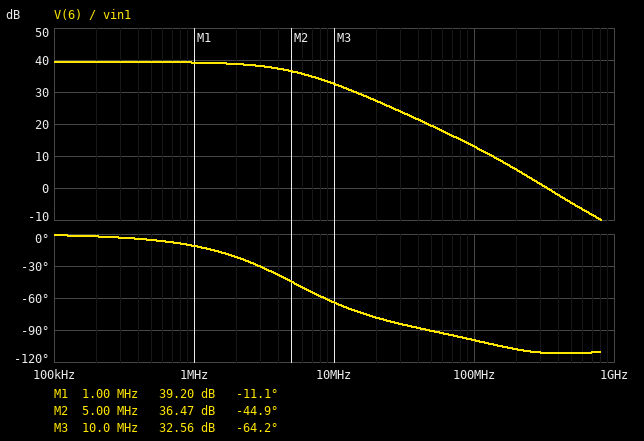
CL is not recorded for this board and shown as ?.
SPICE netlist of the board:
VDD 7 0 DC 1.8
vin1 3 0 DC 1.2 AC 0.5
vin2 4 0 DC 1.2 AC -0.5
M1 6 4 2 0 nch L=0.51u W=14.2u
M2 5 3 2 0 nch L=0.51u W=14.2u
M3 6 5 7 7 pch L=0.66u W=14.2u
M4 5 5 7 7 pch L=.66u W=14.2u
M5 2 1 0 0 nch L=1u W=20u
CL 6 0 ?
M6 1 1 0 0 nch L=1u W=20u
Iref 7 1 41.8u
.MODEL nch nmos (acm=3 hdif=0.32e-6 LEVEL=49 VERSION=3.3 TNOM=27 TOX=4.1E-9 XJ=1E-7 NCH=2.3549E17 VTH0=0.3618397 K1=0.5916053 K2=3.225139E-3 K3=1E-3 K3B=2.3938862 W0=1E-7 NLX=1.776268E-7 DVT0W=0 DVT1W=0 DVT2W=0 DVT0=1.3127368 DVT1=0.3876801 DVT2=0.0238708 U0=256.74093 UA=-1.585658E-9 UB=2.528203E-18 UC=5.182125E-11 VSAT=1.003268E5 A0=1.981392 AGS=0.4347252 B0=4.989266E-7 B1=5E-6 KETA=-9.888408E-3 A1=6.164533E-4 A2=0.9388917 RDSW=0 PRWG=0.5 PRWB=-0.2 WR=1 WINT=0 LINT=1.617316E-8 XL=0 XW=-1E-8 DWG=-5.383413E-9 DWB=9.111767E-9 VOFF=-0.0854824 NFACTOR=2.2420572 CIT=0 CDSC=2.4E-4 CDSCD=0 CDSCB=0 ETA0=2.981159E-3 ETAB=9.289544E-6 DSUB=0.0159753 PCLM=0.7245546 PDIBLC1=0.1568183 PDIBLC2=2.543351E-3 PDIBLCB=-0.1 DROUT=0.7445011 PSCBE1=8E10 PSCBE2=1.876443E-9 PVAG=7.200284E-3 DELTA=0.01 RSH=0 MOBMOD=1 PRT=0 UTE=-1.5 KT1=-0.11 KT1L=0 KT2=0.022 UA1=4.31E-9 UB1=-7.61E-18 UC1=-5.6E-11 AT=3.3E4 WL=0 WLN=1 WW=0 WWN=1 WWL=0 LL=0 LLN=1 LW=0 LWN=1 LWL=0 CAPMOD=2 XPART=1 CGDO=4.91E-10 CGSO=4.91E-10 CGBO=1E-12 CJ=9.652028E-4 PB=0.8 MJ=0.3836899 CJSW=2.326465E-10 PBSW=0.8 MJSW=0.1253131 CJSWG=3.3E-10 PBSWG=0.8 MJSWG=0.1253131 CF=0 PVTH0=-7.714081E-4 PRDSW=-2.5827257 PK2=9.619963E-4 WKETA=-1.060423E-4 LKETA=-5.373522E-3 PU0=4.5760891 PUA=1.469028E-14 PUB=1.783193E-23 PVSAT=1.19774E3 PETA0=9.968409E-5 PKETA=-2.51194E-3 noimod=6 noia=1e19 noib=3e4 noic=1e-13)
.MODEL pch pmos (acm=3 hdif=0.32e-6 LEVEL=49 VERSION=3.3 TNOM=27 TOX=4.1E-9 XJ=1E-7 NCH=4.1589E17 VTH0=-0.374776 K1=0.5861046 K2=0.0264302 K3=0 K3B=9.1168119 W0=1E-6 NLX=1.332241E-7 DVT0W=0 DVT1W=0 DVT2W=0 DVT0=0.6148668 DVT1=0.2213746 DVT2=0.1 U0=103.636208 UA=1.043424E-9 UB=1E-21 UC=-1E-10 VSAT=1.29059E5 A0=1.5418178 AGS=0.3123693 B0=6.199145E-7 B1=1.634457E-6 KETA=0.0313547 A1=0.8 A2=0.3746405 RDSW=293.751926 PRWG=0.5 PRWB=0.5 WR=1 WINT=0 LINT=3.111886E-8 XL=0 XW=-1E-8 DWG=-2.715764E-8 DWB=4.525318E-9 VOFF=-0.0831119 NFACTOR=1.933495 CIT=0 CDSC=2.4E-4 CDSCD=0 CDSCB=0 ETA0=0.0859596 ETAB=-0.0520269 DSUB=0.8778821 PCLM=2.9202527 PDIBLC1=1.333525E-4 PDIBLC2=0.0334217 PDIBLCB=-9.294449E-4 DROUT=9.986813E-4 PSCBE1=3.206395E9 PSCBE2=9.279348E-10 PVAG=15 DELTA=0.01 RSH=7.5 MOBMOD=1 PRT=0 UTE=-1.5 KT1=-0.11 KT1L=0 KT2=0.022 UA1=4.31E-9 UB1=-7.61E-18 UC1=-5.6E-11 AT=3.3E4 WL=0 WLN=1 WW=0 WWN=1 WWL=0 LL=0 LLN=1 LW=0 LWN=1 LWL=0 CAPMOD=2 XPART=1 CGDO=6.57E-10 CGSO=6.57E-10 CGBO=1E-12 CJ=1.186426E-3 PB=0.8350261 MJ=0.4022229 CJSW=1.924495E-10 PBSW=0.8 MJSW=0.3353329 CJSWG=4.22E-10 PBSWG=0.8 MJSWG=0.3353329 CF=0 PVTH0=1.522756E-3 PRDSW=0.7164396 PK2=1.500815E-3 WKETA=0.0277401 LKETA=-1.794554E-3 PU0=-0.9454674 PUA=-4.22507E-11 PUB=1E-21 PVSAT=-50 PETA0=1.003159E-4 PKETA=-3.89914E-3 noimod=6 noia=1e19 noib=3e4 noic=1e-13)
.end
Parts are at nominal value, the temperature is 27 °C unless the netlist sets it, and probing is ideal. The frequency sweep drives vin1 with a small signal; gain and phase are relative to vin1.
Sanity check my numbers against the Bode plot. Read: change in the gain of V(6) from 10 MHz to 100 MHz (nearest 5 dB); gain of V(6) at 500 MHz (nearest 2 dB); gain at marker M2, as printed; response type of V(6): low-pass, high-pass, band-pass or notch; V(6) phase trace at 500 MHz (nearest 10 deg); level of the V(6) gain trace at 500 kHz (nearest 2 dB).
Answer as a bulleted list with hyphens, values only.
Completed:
- -20 dB
- -4 dB
- 36.47 dB
- low-pass
- -110 deg
- 40 dB
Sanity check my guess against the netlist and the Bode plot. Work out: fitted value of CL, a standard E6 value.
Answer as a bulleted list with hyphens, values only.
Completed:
- 150 fF
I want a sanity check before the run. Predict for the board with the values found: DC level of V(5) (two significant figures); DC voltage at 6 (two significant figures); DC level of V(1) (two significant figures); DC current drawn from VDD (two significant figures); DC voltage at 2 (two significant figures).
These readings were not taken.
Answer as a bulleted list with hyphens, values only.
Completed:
- 1.2 V
- 1.2 V
- 550 mV
- 84 µA
- 550 mV
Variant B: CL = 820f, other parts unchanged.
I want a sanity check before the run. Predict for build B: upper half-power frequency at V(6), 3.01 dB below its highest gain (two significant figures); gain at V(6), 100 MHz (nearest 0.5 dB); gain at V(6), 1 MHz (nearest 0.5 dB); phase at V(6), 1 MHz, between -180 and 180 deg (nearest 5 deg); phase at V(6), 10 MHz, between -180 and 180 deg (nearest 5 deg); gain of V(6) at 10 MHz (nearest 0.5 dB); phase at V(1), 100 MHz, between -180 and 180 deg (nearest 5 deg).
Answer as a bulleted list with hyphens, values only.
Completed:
- 1.2 MHz
- 0.5 dB
- 37.0 dB
- -40 deg
- -85 deg
- 21.0 dB
- 70 deg
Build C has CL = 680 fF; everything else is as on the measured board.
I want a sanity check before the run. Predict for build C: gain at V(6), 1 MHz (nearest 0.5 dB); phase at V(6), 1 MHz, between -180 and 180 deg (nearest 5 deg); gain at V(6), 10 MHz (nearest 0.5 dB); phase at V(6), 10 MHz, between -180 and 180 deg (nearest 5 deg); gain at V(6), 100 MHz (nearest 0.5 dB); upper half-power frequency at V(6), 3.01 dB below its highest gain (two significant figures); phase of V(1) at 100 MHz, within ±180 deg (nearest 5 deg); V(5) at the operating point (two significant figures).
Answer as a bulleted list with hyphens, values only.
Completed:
- 37.5 dB
- -35 deg
- 22.5 dB
- -85 deg
- 2.0 dB
- 1.4 MHz
- 70 deg
- 1.2 V
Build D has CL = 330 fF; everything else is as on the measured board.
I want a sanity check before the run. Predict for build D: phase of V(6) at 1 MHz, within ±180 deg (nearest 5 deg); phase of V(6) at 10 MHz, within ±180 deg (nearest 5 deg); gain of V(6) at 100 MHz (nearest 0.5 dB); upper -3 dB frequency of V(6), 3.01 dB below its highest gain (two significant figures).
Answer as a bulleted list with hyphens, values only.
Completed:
- -20 deg
- -75 deg
- 7.5 dB
- 2.7 MHz
